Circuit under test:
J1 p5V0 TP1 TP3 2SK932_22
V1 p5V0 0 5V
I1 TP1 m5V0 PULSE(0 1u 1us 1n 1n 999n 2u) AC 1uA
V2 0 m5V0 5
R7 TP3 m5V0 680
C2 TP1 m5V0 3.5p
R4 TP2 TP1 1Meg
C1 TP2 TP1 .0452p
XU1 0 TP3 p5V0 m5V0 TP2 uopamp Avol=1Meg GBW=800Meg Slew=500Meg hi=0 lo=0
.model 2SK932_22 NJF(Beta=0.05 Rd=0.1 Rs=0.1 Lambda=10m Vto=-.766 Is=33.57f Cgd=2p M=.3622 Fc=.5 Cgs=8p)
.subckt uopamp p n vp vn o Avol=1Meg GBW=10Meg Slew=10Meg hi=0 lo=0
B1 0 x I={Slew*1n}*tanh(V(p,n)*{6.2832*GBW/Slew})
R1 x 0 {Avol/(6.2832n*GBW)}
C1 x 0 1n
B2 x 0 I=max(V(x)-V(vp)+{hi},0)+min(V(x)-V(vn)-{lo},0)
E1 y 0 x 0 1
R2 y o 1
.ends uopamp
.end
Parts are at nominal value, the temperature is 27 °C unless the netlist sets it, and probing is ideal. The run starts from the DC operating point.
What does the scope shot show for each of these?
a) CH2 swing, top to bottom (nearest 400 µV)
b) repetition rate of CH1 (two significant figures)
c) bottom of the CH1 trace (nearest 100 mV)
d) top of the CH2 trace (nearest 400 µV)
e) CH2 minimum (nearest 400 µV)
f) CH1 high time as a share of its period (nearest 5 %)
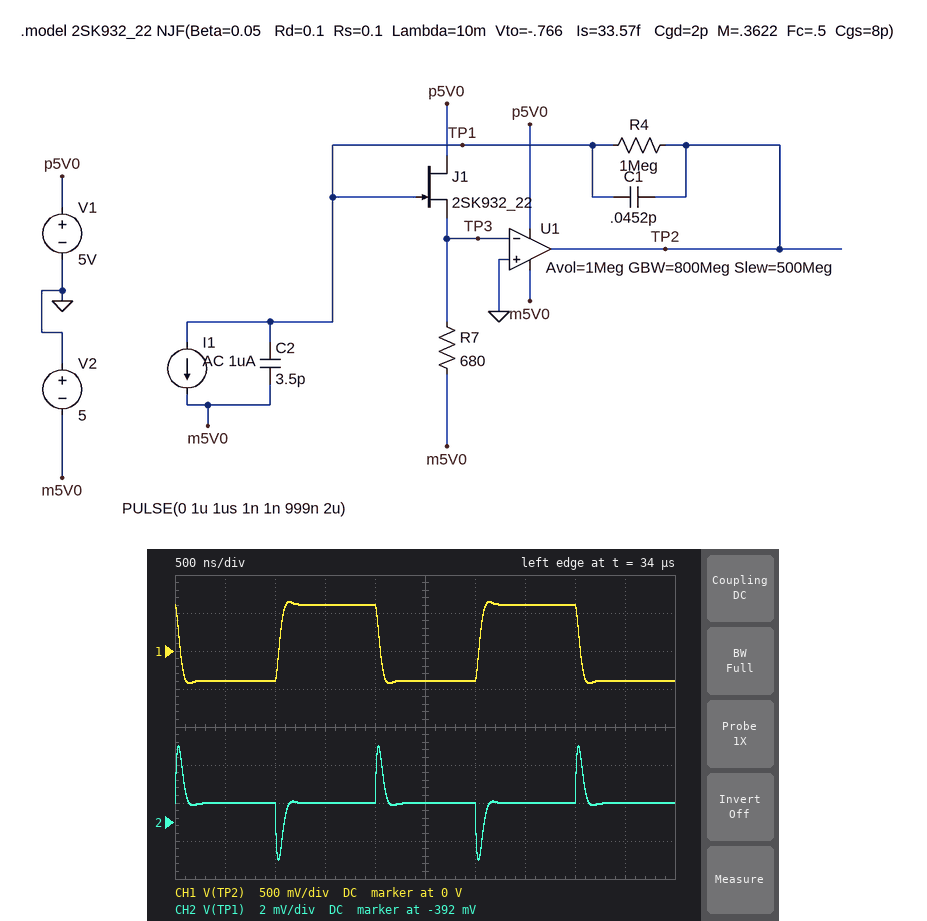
6.0 mV
500 kHz
-400 mV
-388.0 mV
-394.0 mV
50 %
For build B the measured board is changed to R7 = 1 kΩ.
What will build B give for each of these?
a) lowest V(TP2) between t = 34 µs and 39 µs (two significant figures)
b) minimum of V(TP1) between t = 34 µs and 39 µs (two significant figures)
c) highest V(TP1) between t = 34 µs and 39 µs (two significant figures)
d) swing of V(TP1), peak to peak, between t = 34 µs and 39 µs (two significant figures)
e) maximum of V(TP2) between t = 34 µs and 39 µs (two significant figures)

-490 mV
-460 mV
-450 mV
6.0 mV
570 mV
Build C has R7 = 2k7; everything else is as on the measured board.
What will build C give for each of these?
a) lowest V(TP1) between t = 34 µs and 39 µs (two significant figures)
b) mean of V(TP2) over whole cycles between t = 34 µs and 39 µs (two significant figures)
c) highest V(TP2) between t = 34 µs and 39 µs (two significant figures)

-580 mV
-78 mV
450 mV
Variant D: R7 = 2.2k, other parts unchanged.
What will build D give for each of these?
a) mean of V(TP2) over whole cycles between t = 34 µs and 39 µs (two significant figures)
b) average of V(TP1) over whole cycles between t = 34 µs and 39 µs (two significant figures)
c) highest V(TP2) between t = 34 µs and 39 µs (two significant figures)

-58 mV
-560 mV
470 mV
